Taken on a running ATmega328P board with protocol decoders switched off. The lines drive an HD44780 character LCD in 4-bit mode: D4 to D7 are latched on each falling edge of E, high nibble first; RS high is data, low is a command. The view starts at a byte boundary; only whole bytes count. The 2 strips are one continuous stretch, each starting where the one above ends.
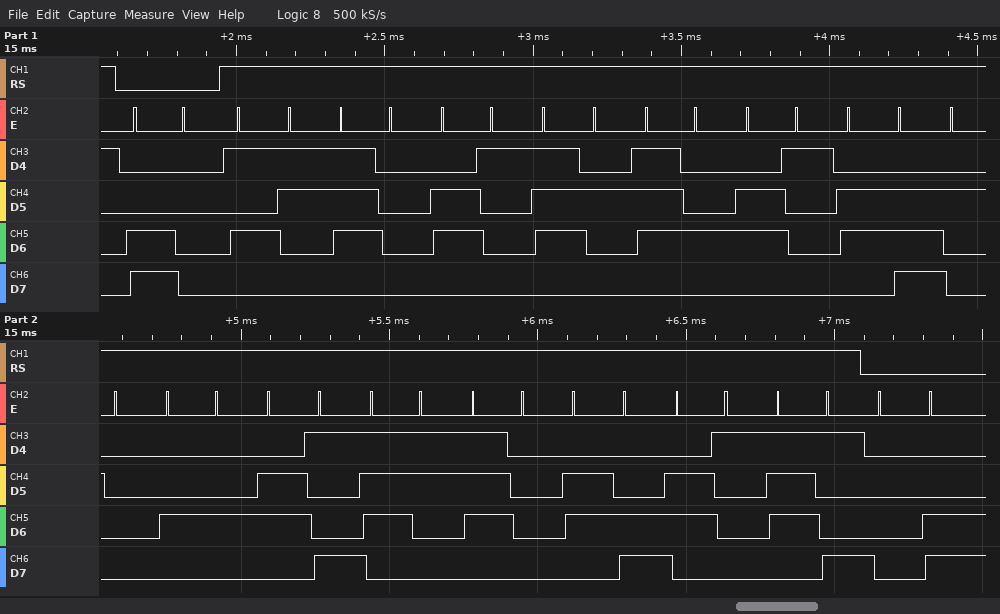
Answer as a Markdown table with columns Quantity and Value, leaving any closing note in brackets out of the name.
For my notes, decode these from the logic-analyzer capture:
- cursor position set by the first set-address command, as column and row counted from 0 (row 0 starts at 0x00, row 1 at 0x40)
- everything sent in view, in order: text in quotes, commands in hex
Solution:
| Quantity | Value |
|---|---|
| cursor position set by the first set-address command, as column and row counted from 0 | column 0, row 1 |
| everything sent in view, in order: text in quotes, commands in hex | 0xC0 "Spartan Display" 0x0C |
